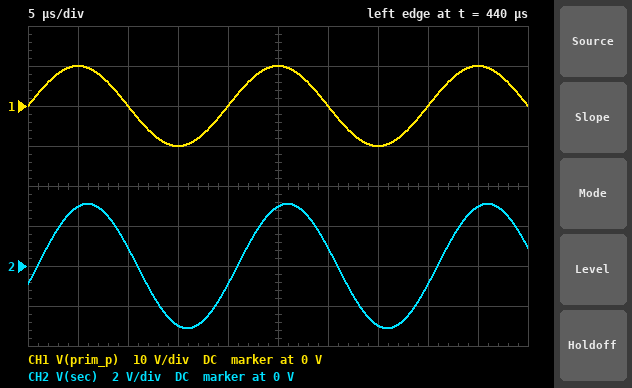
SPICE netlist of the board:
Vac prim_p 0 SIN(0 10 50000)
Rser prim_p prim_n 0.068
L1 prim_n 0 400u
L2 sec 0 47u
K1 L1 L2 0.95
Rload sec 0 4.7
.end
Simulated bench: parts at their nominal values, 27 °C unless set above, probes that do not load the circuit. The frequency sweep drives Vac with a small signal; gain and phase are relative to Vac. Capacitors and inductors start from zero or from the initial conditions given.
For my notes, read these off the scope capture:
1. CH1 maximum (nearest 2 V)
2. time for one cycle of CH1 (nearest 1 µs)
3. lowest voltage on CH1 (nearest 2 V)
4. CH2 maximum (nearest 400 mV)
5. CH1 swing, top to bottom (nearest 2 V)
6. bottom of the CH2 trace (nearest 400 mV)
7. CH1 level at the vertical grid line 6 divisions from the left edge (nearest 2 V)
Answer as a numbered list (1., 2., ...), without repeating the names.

1. 10 V
2. 20 µs
3. -10 V
4. 3.2 V
5. 20 V
6. -3.2 V
7. 0 V
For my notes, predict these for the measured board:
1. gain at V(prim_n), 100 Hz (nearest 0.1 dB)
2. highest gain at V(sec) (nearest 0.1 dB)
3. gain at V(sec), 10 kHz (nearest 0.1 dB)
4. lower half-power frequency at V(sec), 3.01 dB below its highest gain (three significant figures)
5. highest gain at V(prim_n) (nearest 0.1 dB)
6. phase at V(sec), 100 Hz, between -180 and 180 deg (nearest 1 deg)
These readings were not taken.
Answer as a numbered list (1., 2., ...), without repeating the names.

1. -0.3 dB
2. -9.8 dB
3. -9.8 dB
4. 27.0 Hz
5. 0 dB
6. 15 deg
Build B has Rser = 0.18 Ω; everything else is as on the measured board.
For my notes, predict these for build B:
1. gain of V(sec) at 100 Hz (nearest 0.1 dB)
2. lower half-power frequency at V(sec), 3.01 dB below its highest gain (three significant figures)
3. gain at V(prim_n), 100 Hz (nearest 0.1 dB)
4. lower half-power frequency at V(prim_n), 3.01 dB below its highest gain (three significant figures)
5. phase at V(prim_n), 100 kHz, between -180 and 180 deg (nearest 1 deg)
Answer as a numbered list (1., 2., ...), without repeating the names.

1. -11.6 dB
2. 71.3 Hz
3. -1.8 dB
4. 71.9 Hz
5. 0 deg
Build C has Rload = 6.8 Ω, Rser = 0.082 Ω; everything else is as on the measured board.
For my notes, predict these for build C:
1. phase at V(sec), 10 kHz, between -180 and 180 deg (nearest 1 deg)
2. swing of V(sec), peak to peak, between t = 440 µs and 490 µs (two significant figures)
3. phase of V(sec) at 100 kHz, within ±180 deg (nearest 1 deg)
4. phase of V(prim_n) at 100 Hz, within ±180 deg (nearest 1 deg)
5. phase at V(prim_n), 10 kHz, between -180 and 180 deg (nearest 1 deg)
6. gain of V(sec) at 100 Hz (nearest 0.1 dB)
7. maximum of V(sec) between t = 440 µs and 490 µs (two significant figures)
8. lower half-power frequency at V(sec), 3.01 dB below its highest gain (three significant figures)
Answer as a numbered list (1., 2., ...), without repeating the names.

1. -2 deg
2. 6.4 V
3. -23 deg
4. 18 deg
5. 0 deg
6. -10.2 dB
7. 3.2 V
8. 32.6 Hz
